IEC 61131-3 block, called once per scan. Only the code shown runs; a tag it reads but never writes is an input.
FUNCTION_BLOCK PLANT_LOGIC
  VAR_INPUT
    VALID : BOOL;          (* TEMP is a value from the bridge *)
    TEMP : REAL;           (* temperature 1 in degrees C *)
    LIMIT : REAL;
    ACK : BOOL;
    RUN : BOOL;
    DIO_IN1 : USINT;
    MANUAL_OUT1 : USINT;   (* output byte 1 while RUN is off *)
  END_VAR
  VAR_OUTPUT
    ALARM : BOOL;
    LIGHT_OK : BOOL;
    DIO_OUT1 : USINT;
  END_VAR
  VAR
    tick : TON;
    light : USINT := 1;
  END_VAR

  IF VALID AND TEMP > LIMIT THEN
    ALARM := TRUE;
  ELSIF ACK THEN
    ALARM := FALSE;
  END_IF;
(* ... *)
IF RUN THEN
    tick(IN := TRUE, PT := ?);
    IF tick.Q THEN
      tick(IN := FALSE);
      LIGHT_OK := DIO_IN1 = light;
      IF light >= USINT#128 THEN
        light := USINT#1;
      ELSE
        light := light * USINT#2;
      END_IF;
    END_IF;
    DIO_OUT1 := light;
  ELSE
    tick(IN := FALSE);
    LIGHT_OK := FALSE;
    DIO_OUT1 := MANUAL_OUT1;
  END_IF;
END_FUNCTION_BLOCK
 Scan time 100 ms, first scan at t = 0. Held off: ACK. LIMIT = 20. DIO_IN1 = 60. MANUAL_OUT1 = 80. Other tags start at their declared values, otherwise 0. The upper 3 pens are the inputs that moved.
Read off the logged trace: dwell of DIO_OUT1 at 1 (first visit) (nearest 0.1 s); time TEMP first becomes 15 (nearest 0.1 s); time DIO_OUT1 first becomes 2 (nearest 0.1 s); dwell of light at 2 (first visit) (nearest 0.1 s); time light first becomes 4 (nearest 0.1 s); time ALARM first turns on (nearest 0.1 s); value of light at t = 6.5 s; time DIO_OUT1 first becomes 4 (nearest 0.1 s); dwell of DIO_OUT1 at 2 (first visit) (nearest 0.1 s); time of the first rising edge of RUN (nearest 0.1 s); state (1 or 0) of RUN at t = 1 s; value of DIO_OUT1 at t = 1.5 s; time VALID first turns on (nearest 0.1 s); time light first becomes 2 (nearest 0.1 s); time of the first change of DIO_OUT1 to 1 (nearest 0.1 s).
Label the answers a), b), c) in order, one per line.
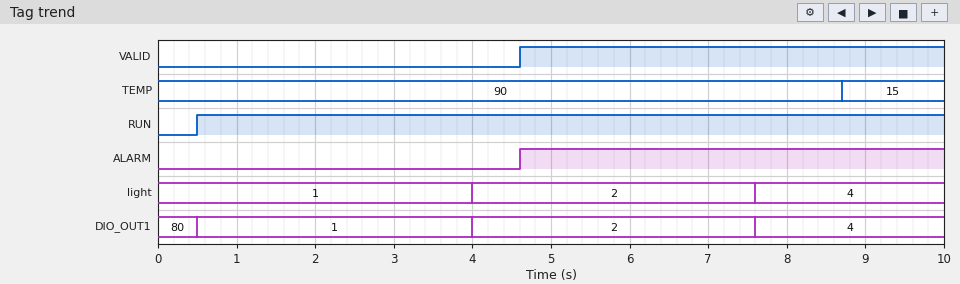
a) 3.5 s
b) 8.7 s
c) 4.0 s
d) 3.6 s
e) 7.6 s
f) 4.6 s
g) 2
h) 7.6 s
i) 3.6 s
j) 0.5 s
k) 1
l) 1
m) 4.6 s
n) 4.0 s
o) 0.5 s
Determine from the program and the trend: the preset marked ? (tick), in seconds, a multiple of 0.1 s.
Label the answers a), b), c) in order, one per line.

a) 3.5 s
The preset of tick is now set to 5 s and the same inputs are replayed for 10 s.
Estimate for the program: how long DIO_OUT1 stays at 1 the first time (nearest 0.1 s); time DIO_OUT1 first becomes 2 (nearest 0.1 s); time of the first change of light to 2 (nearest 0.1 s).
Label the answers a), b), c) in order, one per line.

a) 5.0 s
b) 5.5 s
c) 5.5 s
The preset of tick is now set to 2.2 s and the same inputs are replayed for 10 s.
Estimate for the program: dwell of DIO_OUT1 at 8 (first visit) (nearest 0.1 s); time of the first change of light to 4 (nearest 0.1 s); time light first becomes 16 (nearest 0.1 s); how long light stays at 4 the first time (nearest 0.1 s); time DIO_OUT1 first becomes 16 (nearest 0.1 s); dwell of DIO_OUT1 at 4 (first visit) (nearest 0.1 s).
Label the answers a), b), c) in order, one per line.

a) 2.3 s
b) 5.0 s
c) 9.6 s
d) 2.3 s
e) 9.6 s
f) 2.3 s
